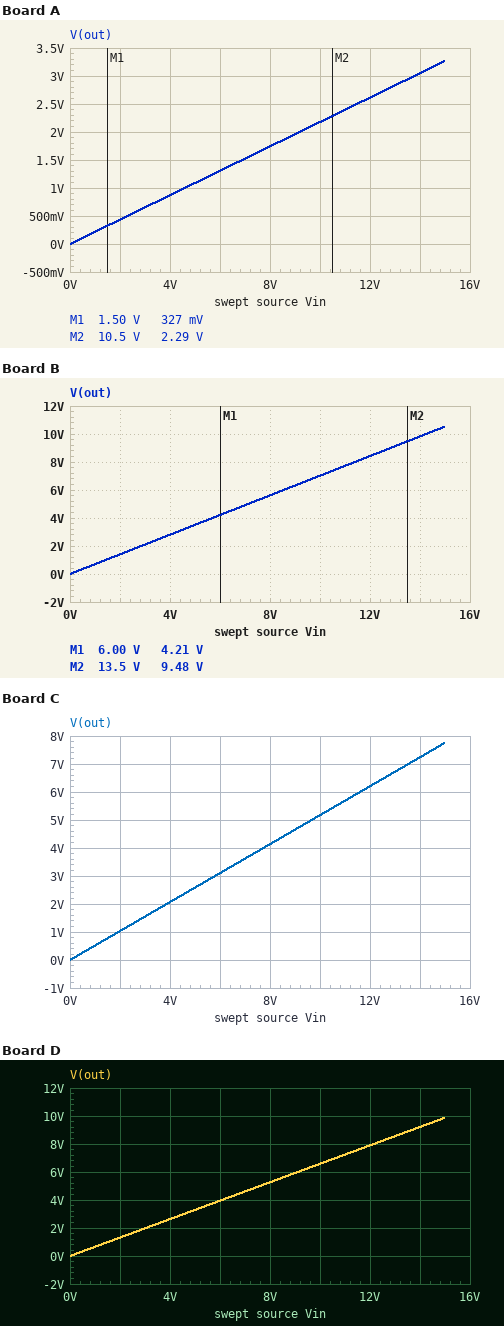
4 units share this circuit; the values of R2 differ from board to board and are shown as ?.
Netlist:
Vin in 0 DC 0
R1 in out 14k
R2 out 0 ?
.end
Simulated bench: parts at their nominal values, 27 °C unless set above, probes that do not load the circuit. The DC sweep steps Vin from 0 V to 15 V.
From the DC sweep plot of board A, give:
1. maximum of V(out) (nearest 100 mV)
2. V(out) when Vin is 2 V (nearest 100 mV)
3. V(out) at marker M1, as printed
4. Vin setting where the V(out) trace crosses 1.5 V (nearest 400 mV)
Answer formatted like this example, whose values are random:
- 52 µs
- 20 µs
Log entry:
- 3.3 V
- 400 mV
- 327 mV
- 6.8 V
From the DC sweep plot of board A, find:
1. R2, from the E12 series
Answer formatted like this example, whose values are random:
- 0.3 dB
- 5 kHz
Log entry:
- 3.9 kΩ
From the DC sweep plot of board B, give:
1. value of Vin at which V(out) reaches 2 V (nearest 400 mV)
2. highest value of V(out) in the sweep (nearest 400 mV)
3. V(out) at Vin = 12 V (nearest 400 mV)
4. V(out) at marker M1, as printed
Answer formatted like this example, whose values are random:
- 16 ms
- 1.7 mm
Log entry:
- 2.8 V
- 10.4 V
- 8.4 V
- 4.21 V
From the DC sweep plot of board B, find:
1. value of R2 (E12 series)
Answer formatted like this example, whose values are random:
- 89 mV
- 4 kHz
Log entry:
- 33 kΩ
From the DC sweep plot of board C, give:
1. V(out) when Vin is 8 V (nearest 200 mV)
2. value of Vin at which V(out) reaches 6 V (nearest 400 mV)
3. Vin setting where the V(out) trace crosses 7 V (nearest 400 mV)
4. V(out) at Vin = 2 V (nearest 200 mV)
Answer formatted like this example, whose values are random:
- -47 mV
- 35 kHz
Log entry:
- 4.2 V
- 11.6 V
- 13.6 V
- 1.0 V
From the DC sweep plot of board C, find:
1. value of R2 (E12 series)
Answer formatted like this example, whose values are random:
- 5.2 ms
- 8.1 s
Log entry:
- 15 kΩ
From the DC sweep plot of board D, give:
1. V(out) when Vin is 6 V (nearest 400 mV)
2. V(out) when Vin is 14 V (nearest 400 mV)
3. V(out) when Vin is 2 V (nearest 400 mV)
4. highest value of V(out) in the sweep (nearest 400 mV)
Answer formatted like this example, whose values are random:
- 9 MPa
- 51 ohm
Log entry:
- 4.0 V
- 9.2 V
- 1.2 V
- 10.0 V
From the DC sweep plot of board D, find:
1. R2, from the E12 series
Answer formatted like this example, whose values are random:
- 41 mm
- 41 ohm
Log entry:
- 27 kΩ
